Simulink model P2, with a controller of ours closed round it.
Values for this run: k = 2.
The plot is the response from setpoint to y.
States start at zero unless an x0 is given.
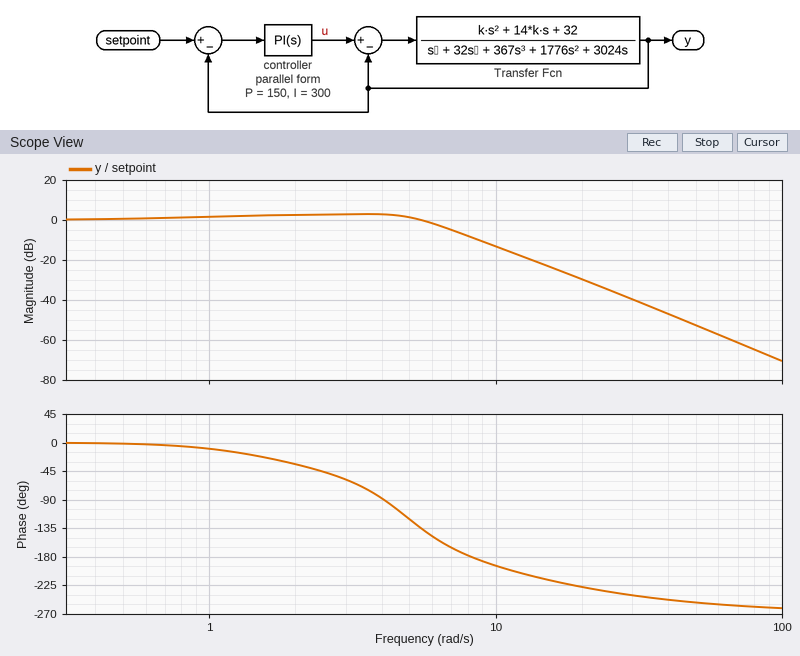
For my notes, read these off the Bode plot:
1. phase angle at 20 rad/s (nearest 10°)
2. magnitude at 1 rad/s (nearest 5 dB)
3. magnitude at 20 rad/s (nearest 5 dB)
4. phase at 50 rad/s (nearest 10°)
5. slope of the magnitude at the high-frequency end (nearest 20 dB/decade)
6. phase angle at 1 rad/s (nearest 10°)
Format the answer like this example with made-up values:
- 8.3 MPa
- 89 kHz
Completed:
- -230°
- 0 dB
- -30 dB
- -250°
- -60 dB/decade
- -10°
